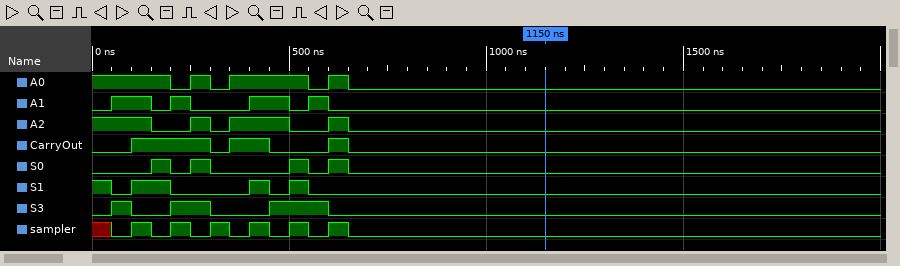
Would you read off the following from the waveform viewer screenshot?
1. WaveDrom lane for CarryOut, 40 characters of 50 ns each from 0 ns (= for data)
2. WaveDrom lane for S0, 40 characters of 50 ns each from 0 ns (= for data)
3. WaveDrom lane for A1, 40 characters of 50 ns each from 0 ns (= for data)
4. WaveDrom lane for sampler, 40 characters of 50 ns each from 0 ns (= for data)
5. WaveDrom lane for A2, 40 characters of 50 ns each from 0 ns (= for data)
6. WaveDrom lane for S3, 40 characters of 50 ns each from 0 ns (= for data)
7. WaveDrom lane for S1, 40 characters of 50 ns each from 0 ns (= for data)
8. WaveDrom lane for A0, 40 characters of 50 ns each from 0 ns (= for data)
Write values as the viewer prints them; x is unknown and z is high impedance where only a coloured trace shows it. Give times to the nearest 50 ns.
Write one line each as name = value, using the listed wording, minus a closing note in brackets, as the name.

WaveDrom lane for CarryOut, 40 characters of 50 ns each from 0 ns = {name: 'CarryOut', wave: '0.1...01.0..10..........................'}
WaveDrom lane for S0, 40 characters of 50 ns each from 0 ns = {name: 'S0', wave: '0..1010...1010..........................'}
WaveDrom lane for A1, 40 characters of 50 ns each from 0 ns = {name: 'A1', wave: '01.010..1.010...........................'}
WaveDrom lane for sampler, 40 characters of 50 ns each from 0 ns = {name: 'sampler', wave: 'x0101010101010..........................'}
WaveDrom lane for A2, 40 characters of 50 ns each from 0 ns = {name: 'A2', wave: '1..0.101..0.10..........................'}
WaveDrom lane for S3, 40 characters of 50 ns each from 0 ns = {name: 'S3', wave: '010.1.0..1..0...........................'}
WaveDrom lane for S1, 40 characters of 50 ns each from 0 ns = {name: 'S1', wave: '101.0...1010............................'}
WaveDrom lane for A0, 40 characters of 50 ns each from 0 ns = {name: 'A0', wave: '1...0101...010..........................'}
